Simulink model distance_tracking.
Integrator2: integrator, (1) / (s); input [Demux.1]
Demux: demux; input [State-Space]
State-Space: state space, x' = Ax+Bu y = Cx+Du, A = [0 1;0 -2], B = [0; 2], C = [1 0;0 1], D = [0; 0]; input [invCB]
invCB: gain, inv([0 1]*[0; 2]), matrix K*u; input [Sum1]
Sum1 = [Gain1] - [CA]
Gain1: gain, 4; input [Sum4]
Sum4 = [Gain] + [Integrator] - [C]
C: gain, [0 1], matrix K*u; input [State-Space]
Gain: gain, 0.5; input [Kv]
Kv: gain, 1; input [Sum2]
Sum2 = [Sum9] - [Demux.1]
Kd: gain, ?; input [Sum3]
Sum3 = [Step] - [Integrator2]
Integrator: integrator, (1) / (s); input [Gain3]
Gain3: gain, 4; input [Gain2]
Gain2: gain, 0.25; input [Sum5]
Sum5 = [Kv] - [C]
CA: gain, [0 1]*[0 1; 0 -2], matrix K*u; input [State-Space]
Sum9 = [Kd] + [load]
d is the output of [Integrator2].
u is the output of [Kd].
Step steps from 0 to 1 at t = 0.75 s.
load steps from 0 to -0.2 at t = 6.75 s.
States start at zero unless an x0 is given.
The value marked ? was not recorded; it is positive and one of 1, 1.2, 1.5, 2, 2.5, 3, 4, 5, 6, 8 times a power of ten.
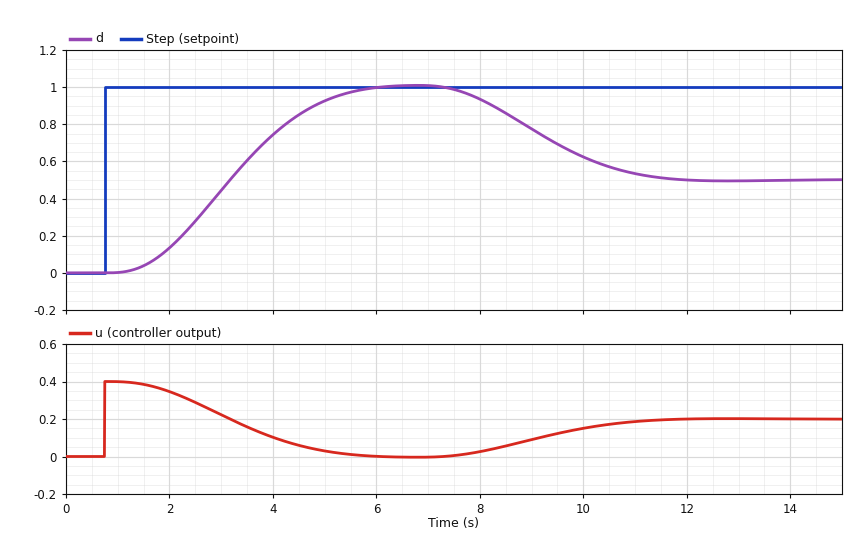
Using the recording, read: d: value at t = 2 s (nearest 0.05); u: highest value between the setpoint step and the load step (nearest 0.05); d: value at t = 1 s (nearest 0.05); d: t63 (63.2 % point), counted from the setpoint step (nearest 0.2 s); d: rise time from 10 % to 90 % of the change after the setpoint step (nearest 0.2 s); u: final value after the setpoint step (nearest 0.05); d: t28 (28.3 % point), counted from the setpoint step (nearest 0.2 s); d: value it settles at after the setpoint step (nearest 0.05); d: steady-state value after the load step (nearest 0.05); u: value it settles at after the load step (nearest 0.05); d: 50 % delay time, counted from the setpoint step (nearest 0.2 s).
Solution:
0.15
0.40
0.00
2.8 s
3.0 s
0.00
1.8 s
1.00
0.50
0.20
2.4 s
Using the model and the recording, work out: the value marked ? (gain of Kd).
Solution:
0.4
